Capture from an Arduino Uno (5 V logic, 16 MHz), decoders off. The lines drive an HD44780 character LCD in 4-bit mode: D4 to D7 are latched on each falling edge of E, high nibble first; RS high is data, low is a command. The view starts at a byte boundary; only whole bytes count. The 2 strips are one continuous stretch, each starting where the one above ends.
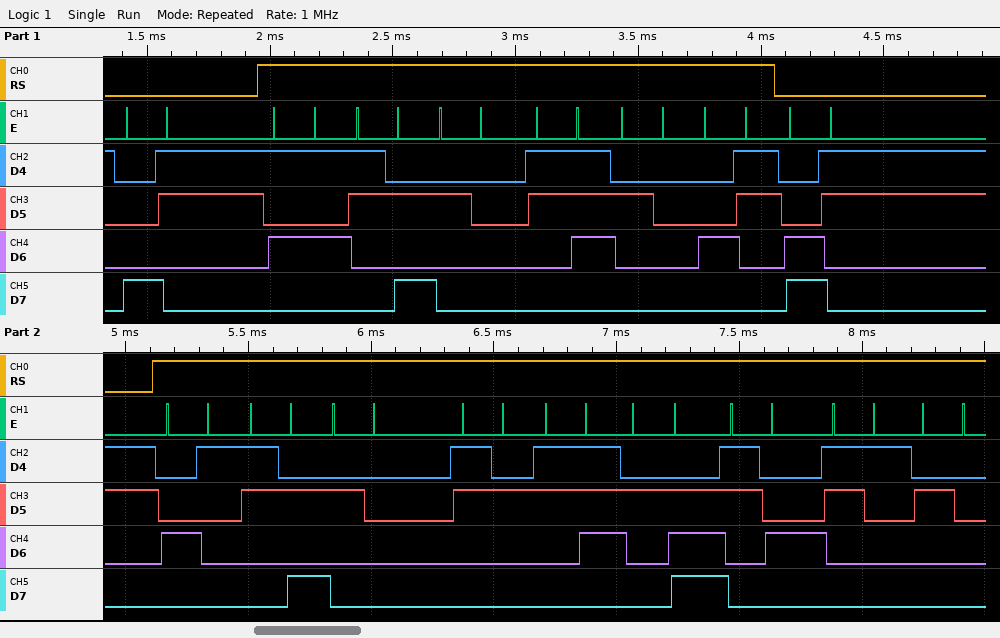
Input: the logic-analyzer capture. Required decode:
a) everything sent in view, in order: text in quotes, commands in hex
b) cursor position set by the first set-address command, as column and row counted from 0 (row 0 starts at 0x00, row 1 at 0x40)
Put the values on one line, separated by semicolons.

0x83 "U: 7 C" 0xC3 "A: 27.41 "; column 3, row 0
